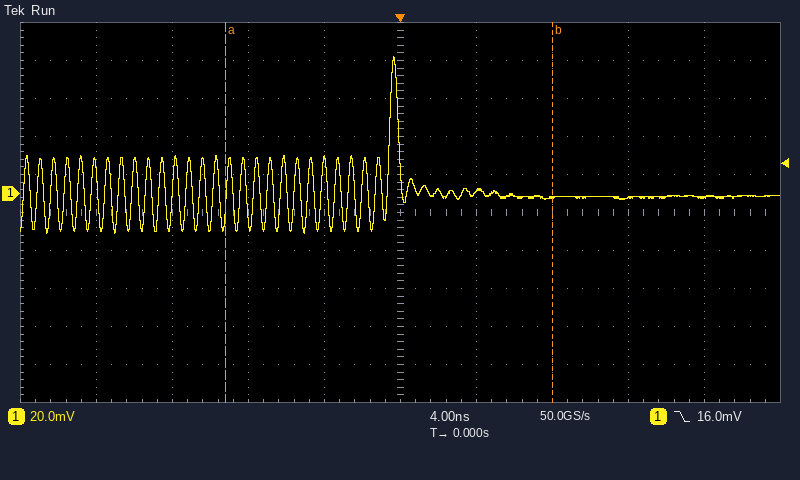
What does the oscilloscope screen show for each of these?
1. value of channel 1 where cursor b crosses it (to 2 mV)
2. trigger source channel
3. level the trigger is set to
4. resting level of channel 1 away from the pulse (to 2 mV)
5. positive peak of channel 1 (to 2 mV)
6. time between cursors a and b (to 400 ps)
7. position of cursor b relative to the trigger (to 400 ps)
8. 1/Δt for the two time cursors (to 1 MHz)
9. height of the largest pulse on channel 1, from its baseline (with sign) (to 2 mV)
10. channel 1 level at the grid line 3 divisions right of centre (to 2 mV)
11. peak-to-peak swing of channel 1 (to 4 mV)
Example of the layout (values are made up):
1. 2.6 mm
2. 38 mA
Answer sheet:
1. -2 mV
2. channel 1
3. 16.0 mV
4. -2 mV
5. 72 mV
6. 17.2 ns
7. +8.0 ns
8. 58 MHz
9. +74 mV
10. -2 mV
11. 92 mV
